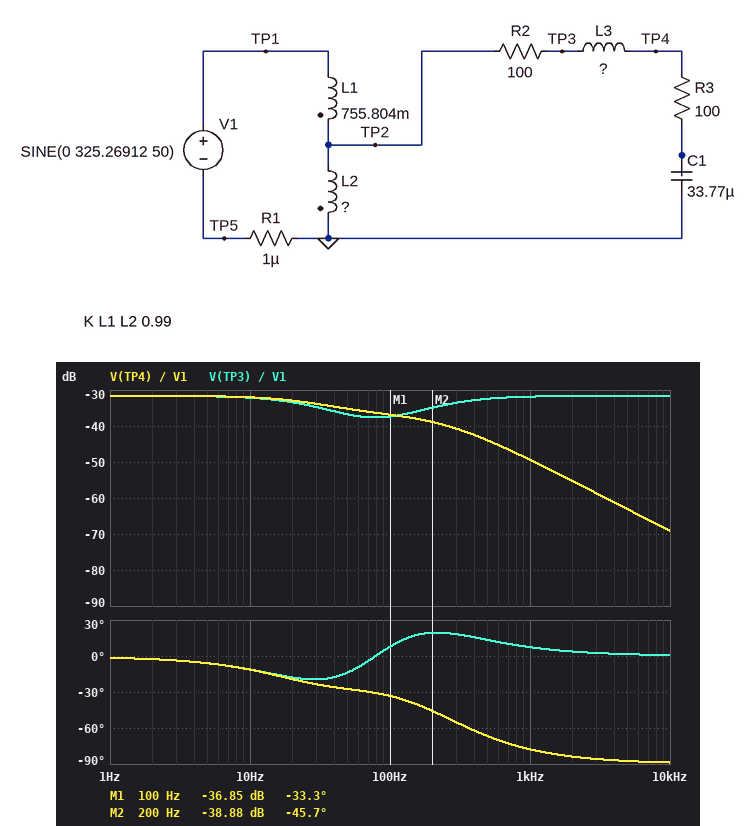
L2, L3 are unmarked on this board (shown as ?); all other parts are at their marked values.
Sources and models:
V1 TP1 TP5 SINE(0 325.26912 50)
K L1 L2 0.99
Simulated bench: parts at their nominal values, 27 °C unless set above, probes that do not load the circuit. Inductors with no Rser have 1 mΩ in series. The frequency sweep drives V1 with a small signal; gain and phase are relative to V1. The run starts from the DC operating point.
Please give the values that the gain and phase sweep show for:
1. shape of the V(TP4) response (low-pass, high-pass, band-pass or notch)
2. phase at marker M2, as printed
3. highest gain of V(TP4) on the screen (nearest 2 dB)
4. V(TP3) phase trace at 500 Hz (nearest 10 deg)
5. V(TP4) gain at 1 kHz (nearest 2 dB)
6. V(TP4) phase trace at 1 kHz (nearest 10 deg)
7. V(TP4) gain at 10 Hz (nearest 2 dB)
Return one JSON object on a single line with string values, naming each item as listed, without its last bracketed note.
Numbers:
{"shape of the V(TP4) response": "low-pass", "phase at marker M2, as printed": "-45.7 deg", "highest gain of V(TP4) on the screen": "-32 dB", "V(TP3) phase trace at 500 Hz": "10 deg", "V(TP4) gain at 1 kHz": "-50 dB", "V(TP4) phase trace at 1 kHz": "-80 deg", "V(TP4) gain at 10 Hz": "-32 dB"}
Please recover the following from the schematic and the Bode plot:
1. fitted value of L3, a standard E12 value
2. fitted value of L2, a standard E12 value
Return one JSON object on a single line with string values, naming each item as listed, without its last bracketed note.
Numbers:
{"fitted value of L3, a standard E12 value": "120 mH", "fitted value of L2, a standard E12 value": "560 µH"}
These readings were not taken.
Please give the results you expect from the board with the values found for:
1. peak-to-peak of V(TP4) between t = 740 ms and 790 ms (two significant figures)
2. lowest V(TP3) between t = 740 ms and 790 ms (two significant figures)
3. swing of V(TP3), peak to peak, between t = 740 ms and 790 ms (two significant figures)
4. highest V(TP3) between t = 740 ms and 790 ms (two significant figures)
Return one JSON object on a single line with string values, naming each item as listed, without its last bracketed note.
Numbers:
{"peak-to-peak of V(TP4) between t = 740 ms and 790 ms": "11 V", "lowest V(TP3) between t = 740 ms and 790 ms": "-4.7 V", "swing of V(TP3), peak to peak, between t = 740 ms and 790 ms": "9.4 V", "highest V(TP3) between t = 740 ms and 790 ms": "4.7 V"}
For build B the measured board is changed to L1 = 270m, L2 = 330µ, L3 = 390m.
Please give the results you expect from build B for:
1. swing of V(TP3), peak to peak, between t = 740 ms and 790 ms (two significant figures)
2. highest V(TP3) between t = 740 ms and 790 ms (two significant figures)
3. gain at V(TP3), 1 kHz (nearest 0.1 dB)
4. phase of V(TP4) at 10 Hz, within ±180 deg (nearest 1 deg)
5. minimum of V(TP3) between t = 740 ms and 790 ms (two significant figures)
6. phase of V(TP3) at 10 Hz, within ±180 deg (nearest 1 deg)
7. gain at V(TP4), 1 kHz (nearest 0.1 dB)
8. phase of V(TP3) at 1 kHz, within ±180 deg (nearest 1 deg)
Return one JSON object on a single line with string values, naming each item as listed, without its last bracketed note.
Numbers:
{"swing of V(TP3), peak to peak, between t = 740 ms and 790 ms": "11 V", "highest V(TP3) between t = 740 ms and 790 ms": "5.6 V", "gain at V(TP3), 1 kHz": "-29.5 dB", "phase of V(TP4) at 10 Hz, within ±180 deg": "-12 deg", "minimum of V(TP3) between t = 740 ms and 790 ms": "-5.6 V", "phase of V(TP3) at 10 Hz, within ±180 deg": "-12 deg", "gain at V(TP4), 1 kHz": "-57.3 dB", "phase of V(TP3) at 1 kHz, within ±180 deg": "2 deg"}
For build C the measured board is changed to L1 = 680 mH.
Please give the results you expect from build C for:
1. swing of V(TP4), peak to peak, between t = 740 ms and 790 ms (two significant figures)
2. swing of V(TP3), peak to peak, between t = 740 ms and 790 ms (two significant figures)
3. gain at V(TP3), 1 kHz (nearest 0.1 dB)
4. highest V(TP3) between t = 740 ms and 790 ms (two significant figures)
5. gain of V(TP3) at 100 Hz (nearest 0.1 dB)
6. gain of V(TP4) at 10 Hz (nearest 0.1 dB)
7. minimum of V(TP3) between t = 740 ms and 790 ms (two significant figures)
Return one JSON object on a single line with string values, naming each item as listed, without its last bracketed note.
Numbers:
{"swing of V(TP4), peak to peak, between t = 740 ms and 790 ms": "12 V", "swing of V(TP3), peak to peak, between t = 740 ms and 790 ms": "9.9 V", "gain at V(TP3), 1 kHz": "-31.4 dB", "highest V(TP3) between t = 740 ms and 790 ms": "5.0 V", "gain of V(TP3) at 100 Hz": "-36.9 dB", "gain of V(TP4) at 10 Hz": "-31.6 dB", "minimum of V(TP3) between t = 740 ms and 790 ms": "-5.0 V"}
